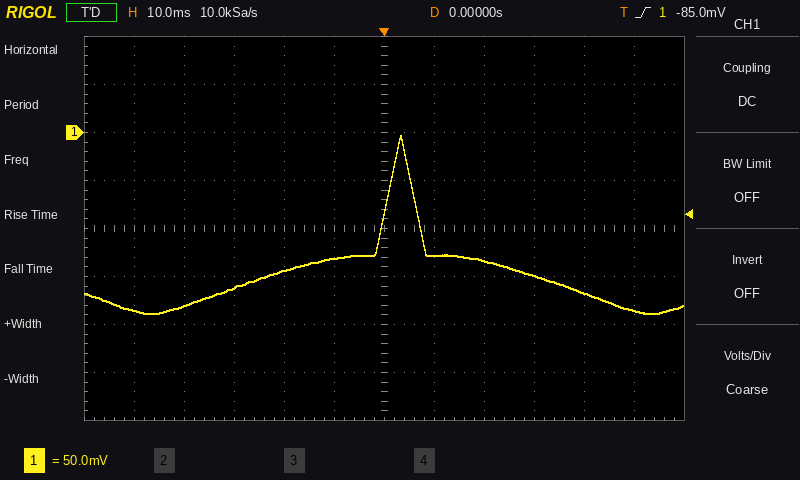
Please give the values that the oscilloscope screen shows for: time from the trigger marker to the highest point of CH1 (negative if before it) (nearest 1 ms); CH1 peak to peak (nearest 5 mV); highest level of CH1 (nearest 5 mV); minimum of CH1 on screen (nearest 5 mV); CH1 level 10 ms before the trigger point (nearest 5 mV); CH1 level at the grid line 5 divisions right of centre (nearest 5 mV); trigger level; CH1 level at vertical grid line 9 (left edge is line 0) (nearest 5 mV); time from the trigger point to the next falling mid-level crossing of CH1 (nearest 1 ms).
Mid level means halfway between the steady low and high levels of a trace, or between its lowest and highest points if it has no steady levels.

+3 ms
185 mV
-5 mV
-190 mV
-130 mV
-185 mV
-85.0 mV
-150 mV
7 ms
